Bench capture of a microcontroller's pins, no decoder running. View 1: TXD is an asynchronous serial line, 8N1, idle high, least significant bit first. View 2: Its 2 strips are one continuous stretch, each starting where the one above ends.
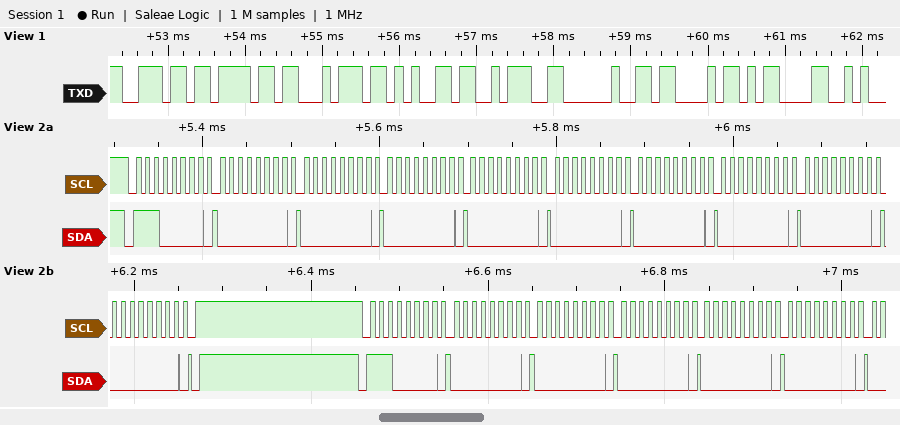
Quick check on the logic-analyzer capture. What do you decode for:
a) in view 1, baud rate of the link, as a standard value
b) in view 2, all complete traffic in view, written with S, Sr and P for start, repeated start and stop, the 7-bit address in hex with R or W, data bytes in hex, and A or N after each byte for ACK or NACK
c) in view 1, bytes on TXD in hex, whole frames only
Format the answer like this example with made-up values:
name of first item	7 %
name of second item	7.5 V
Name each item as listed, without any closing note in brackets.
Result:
in view 1, baud rate of the link, as a standard value	9600 baud
in view 2, all complete traffic in view, written with S, Sr and P for start, repeated start and stop, the 7-bit address in hex with R or W, data bytes in hex, and A or N after each byte for ACK or NACK	S 70W A 00 A 00 A 00 A 00 A 00 A 00 A 00 A 00 A 00 A P S 70W A 00 A 00 A 00 A 00 A 00 A
in view 1, bytes on TXD in hex, whole frames only	0x6E 0x6F 0x74 0x65 0x3A 0x20 0x43 0x0D
